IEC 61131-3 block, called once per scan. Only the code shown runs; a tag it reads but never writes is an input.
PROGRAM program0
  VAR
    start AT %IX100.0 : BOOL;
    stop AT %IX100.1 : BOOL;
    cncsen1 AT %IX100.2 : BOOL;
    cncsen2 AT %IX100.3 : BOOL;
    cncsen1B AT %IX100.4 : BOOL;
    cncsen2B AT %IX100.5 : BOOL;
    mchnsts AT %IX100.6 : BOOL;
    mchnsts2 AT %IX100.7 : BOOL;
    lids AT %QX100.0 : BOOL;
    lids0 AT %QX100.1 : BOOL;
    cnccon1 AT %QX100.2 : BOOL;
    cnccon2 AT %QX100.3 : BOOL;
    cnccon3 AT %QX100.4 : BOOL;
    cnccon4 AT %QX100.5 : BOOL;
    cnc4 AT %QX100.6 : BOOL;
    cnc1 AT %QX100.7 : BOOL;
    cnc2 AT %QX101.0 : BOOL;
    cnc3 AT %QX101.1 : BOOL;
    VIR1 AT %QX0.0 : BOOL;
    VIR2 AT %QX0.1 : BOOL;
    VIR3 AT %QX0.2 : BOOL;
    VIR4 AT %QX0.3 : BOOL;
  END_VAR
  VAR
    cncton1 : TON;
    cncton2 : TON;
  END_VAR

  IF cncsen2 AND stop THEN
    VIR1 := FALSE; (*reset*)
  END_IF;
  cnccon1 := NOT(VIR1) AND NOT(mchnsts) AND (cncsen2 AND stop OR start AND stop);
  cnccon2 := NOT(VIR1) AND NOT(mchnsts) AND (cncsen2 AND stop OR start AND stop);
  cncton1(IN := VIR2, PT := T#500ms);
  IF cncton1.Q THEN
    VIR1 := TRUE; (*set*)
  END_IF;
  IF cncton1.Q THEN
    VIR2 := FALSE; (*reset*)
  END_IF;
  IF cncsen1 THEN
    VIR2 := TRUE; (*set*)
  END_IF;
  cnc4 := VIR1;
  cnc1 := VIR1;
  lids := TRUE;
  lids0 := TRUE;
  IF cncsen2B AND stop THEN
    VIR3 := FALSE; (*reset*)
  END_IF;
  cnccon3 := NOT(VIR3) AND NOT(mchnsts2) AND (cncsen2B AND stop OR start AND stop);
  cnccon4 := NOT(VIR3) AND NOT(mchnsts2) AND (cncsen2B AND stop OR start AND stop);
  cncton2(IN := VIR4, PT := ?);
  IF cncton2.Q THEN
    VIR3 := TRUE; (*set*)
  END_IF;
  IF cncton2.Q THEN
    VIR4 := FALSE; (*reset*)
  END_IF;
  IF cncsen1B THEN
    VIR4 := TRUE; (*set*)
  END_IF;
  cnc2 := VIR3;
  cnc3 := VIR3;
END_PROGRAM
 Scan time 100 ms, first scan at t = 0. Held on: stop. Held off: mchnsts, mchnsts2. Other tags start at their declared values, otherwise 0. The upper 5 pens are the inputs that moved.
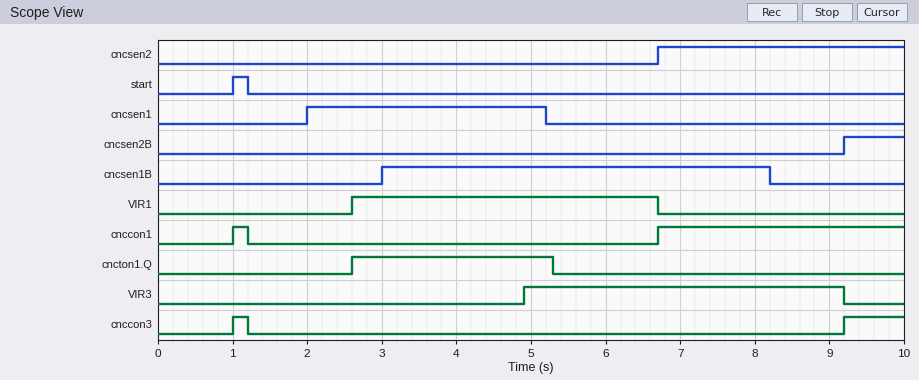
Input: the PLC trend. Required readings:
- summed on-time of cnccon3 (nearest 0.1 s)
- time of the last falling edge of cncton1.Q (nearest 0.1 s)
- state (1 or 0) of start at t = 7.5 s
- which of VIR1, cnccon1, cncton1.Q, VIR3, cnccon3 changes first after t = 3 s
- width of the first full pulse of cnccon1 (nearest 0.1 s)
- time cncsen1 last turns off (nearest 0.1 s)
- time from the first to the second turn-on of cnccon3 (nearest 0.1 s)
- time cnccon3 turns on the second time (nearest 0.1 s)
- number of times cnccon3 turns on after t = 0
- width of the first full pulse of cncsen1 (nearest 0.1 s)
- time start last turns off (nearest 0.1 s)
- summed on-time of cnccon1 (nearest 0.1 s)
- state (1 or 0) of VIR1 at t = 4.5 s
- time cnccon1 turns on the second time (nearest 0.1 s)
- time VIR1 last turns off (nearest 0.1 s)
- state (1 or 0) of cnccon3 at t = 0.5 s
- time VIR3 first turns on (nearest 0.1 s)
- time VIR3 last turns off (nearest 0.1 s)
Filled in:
1.0 s
5.3 s
0
VIR3
0.2 s
5.2 s
8.2 s
9.2 s
2
3.2 s
1.2 s
3.5 s
1
6.7 s
6.7 s
0
4.9 s
9.2 s
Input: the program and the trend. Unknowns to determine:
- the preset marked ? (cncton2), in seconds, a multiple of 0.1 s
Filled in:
1.8 s
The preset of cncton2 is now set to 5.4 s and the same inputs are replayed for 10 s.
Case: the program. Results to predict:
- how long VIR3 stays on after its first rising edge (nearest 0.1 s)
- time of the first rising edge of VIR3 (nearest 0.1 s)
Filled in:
0.7 s
8.5 s
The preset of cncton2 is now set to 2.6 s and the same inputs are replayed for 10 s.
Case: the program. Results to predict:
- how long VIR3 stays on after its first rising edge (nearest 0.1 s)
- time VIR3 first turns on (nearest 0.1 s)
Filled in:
3.5 s
5.7 s
